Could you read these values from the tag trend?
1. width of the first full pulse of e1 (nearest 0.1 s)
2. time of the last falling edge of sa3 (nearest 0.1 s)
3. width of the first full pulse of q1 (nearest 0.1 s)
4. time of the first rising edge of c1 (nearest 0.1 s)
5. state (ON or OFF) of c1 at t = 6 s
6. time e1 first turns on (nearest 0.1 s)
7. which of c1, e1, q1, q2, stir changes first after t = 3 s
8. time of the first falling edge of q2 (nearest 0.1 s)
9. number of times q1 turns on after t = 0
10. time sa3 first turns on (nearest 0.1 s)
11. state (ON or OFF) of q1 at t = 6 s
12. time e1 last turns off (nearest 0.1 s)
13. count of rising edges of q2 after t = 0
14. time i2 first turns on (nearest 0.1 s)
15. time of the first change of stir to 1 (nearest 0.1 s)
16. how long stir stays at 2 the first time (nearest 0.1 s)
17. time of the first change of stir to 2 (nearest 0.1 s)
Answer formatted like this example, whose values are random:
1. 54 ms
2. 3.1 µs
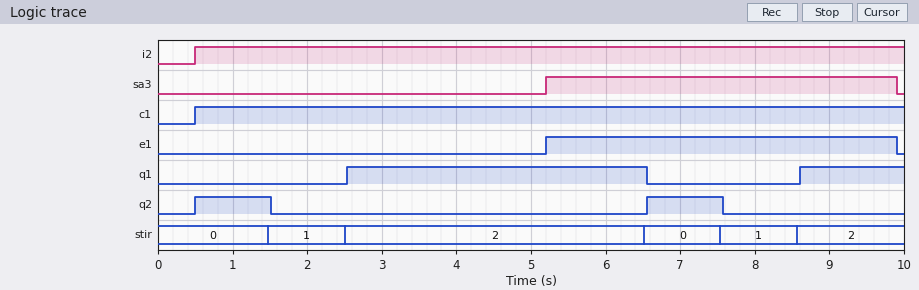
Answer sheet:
1. 4.7 s
2. 9.9 s
3. 4.0 s
4. 0.5 s
5. ON
6. 5.2 s
7. e1
8. 1.5 s
9. 2
10. 5.2 s
11. ON
12. 9.9 s
13. 2
14. 0.5 s
15. 1.5 s
16. 4.0 s
17. 2.5 s
